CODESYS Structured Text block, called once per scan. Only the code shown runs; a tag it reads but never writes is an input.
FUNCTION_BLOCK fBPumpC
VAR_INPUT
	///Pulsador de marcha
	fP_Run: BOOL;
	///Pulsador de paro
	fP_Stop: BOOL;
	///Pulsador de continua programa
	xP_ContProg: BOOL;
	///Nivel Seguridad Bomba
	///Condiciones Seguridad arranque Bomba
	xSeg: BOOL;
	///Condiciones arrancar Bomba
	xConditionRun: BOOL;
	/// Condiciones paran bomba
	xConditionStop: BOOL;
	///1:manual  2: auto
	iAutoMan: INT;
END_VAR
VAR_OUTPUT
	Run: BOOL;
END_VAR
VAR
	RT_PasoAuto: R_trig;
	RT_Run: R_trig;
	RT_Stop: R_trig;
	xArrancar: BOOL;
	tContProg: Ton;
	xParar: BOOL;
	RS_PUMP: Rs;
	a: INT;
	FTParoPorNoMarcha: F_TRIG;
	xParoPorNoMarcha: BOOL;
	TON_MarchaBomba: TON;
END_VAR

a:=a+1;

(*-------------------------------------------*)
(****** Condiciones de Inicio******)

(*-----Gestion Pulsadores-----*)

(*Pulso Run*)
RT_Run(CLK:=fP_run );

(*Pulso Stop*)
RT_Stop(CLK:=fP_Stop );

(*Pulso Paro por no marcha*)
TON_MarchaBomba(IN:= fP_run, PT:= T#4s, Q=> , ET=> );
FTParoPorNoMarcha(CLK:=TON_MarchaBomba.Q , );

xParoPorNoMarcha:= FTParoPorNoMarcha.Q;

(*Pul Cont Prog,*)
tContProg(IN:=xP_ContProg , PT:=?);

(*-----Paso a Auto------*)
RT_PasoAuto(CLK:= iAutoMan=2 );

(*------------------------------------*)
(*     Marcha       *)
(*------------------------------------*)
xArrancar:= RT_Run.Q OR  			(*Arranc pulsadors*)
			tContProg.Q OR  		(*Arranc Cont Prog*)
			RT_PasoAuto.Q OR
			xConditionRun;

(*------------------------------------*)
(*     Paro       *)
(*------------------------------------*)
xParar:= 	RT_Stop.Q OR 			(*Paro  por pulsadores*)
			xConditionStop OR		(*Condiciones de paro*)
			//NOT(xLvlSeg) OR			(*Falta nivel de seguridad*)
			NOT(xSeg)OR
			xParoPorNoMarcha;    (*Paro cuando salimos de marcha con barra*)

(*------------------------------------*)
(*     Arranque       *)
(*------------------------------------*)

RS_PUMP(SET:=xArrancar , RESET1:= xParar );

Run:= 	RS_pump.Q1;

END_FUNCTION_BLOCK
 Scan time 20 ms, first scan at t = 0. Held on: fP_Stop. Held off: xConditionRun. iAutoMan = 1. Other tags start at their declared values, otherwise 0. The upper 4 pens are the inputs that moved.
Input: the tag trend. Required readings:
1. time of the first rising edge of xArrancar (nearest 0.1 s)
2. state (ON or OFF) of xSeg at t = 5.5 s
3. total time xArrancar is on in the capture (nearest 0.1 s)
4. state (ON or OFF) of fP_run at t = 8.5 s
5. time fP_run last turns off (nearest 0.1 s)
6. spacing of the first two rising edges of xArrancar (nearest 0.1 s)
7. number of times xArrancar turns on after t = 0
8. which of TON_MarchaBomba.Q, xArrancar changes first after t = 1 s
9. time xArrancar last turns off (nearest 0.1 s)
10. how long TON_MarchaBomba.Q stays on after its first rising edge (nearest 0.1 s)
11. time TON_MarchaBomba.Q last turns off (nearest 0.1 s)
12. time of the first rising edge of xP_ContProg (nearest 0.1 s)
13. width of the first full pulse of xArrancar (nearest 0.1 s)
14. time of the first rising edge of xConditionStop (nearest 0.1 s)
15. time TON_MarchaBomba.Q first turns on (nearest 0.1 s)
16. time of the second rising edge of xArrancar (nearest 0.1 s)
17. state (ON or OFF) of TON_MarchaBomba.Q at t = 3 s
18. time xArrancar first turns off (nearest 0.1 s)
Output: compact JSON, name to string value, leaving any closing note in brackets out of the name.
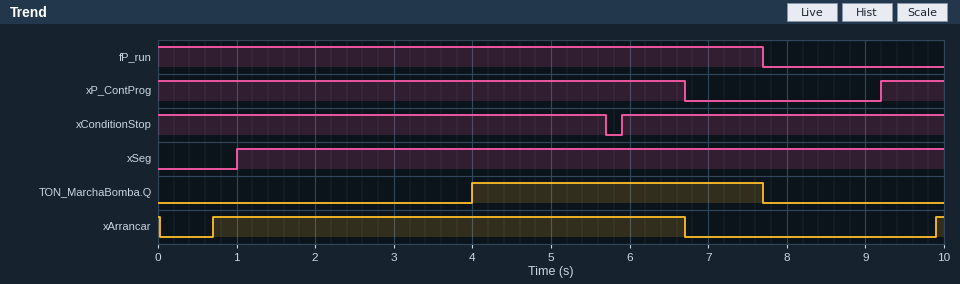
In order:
{"time of the first rising edge of xArrancar": "0.7 s", "state (ON or OFF) of xSeg at t = 5.5 s": "ON", "total time xArrancar is on in the capture": "6.1 s", "state (ON or OFF) of fP_run at t = 8.5 s": "OFF", "time fP_run last turns off": "7.7 s", "spacing of the first two rising edges of xArrancar": "9.2 s", "number of times xArrancar turns on after t = 0": "2", "which of TON_MarchaBomba.Q, xArrancar changes first after t = 1 s": "TON_MarchaBomba.Q", "time xArrancar last turns off": "6.7 s", "how long TON_MarchaBomba.Q stays on after its first rising edge": "3.7 s", "time TON_MarchaBomba.Q last turns off": "7.7 s", "time of the first rising edge of xP_ContProg": "9.2 s", "width of the first full pulse of xArrancar": "6.0 s", "time of the first rising edge of xConditionStop": "5.9 s", "time TON_MarchaBomba.Q first turns on": "4.0 s", "time of the second rising edge of xArrancar": "9.9 s", "state (ON or OFF) of TON_MarchaBomba.Q at t = 3 s": "OFF", "time xArrancar first turns off": "0.0 s"}
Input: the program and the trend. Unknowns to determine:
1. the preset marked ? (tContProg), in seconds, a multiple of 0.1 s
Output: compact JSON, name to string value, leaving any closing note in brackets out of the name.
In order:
{"the preset marked ? (tContProg), in seconds, a multiple of 0.1 s": "0.7 s"}
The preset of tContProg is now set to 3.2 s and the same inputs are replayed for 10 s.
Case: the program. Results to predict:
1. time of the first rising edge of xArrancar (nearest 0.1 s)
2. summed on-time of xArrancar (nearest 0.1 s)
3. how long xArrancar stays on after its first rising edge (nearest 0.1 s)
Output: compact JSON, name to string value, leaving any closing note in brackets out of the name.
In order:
{"time of the first rising edge of xArrancar": "3.2 s", "summed on-time of xArrancar": "3.5 s", "how long xArrancar stays on after its first rising edge": "3.5 s"}
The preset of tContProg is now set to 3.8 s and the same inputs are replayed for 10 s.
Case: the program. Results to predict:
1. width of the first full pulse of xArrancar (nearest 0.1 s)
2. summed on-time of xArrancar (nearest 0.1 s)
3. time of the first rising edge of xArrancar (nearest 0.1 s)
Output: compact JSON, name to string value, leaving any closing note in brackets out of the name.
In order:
{"width of the first full pulse of xArrancar": "2.9 s", "summed on-time of xArrancar": "2.9 s", "time of the first rising edge of xArrancar": "3.8 s"}
